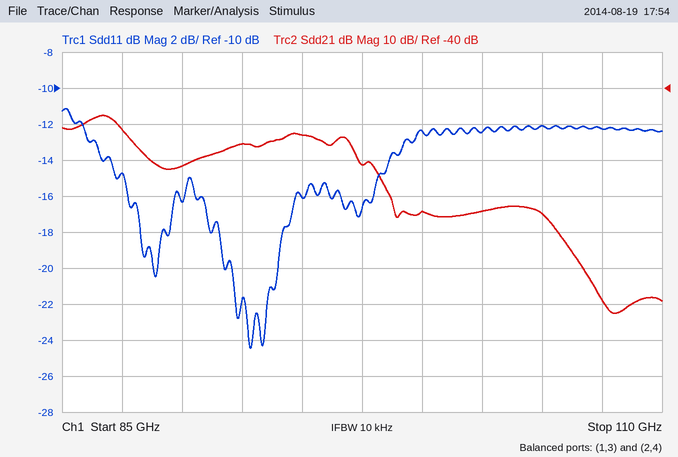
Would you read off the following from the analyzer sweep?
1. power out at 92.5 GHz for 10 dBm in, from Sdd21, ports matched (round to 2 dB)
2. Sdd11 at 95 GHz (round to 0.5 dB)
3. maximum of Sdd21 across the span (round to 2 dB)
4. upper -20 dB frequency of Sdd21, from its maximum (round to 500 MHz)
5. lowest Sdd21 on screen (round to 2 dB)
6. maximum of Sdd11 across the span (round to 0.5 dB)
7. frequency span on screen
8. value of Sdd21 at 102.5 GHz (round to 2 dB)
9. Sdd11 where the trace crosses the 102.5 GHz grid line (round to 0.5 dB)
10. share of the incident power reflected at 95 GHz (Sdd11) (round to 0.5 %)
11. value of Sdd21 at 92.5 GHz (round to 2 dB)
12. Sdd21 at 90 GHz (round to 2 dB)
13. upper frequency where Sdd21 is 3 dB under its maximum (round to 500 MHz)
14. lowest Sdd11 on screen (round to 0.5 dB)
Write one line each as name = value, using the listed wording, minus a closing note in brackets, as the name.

power out at 92.5 GHz for 10 dBm in, from Sdd21, ports matched = -46 dBm
Sdd11 at 95 GHz = -16.0 dB
maximum of Sdd21 across the span = -48 dB
upper -20 dB frequency of Sdd21, from its maximum = 98.5 GHz
lowest Sdd21 on screen = -102 dB
maximum of Sdd11 across the span = -11.0 dB
frequency span on screen = 25 GHz
value of Sdd21 at 102.5 GHz = -74 dB
Sdd11 where the trace crosses the 102.5 GHz grid line = -12.5 dB
share of the incident power reflected at 95 GHz (Sdd11) = 2.5 %
value of Sdd21 at 92.5 GHz = -56 dB
Sdd21 at 90 GHz = -62 dB
upper frequency where Sdd21 is 3 dB under its maximum = 87.5 GHz
lowest Sdd11 on screen = -24.5 dB
